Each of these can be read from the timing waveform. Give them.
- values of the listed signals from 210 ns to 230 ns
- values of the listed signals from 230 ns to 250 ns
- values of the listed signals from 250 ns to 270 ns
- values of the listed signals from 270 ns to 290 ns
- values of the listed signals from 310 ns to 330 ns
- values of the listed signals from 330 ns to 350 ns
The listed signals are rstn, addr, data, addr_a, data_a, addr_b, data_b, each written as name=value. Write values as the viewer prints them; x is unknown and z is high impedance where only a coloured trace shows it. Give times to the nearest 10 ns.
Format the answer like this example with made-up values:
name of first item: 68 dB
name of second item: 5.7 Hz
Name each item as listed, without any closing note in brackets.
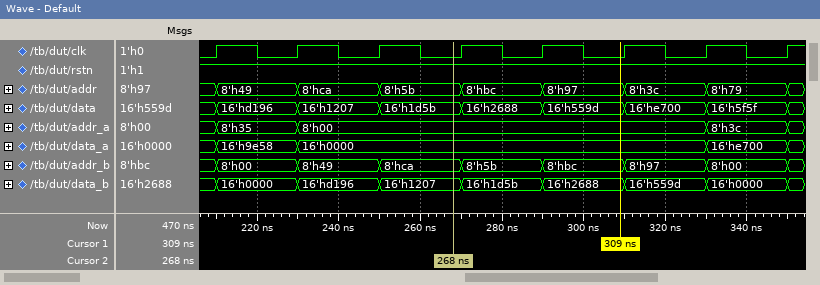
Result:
values of the listed signals from 210 ns to 230 ns: rstn=1, addr=8'h49, data=16'hd196, addr_a=8'h35, data_a=16'h9e58, addr_b=8'h00, data_b=16'h0000
values of the listed signals from 230 ns to 250 ns: rstn=1, addr=8'hca, data=16'h1207, addr_a=8'h00, data_a=16'h0000, addr_b=8'h49, data_b=16'hd196
values of the listed signals from 250 ns to 270 ns: rstn=1, addr=8'h5b, data=16'h1d5b, addr_a=8'h00, data_a=16'h0000, addr_b=8'hca, data_b=16'h1207
values of the listed signals from 270 ns to 290 ns: rstn=1, addr=8'hbc, data=16'h2688, addr_a=8'h00, data_a=16'h0000, addr_b=8'h5b, data_b=16'h1d5b
values of the listed signals from 310 ns to 330 ns: rstn=1, addr=8'h3c, data=16'he700, addr_a=8'h00, data_a=16'h0000, addr_b=8'h97, data_b=16'h559d
values of the listed signals from 330 ns to 350 ns: rstn=1, addr=8'h79, data=16'h5f5f, addr_a=8'h3c, data_a=16'he700, addr_b=8'h00, data_b=16'h0000
